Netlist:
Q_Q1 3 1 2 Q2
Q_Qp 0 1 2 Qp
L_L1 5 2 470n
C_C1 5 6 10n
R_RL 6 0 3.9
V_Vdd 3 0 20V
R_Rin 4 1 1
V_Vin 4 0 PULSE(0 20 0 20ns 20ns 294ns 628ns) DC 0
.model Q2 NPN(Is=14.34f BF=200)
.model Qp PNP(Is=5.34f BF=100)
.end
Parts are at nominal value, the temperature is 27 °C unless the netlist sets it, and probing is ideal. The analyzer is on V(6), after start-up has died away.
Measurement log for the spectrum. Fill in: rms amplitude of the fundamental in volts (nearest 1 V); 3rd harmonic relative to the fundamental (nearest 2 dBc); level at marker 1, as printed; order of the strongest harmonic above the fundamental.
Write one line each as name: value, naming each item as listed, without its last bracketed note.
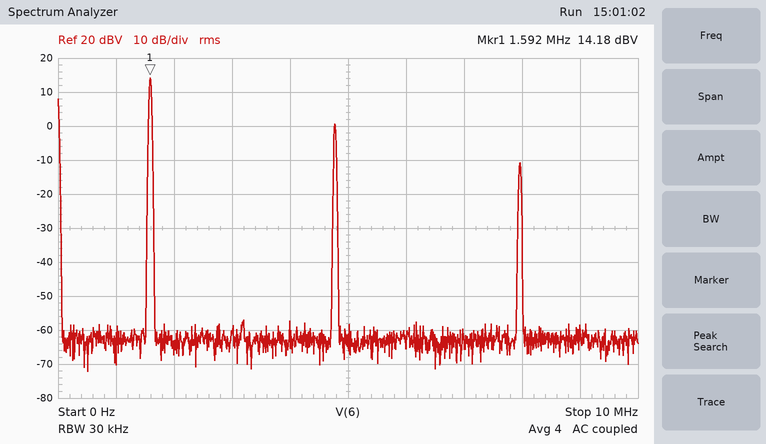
rms amplitude of the fundamental in volts: 5 V
3rd harmonic relative to the fundamental: -14 dBc
level at marker 1, as printed: 14.18 dBV
order of the strongest harmonic above the fundamental: 3
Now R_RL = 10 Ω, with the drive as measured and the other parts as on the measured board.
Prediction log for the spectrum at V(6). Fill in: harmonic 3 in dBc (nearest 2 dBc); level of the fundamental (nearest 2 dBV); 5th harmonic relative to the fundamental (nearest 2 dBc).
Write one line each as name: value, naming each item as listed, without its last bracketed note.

harmonic 3 in dBc: -12 dBc
level of the fundamental: 18 dBV
5th harmonic relative to the fundamental: -20 dBc
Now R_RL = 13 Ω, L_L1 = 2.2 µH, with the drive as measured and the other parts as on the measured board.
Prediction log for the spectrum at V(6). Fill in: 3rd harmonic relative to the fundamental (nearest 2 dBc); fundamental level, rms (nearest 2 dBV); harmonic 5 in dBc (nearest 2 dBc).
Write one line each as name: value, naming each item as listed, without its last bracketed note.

3rd harmonic relative to the fundamental: -20 dBc
fundamental level, rms: 16 dBV
harmonic 5 in dBc: -28 dBc
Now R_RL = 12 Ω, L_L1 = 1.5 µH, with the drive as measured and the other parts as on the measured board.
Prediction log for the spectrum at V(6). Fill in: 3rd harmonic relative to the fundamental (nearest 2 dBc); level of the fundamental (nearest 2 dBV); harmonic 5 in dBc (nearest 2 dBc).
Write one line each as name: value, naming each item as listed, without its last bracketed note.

3rd harmonic relative to the fundamental: -20 dBc
level of the fundamental: 18 dBV
harmonic 5 in dBc: -28 dBc
